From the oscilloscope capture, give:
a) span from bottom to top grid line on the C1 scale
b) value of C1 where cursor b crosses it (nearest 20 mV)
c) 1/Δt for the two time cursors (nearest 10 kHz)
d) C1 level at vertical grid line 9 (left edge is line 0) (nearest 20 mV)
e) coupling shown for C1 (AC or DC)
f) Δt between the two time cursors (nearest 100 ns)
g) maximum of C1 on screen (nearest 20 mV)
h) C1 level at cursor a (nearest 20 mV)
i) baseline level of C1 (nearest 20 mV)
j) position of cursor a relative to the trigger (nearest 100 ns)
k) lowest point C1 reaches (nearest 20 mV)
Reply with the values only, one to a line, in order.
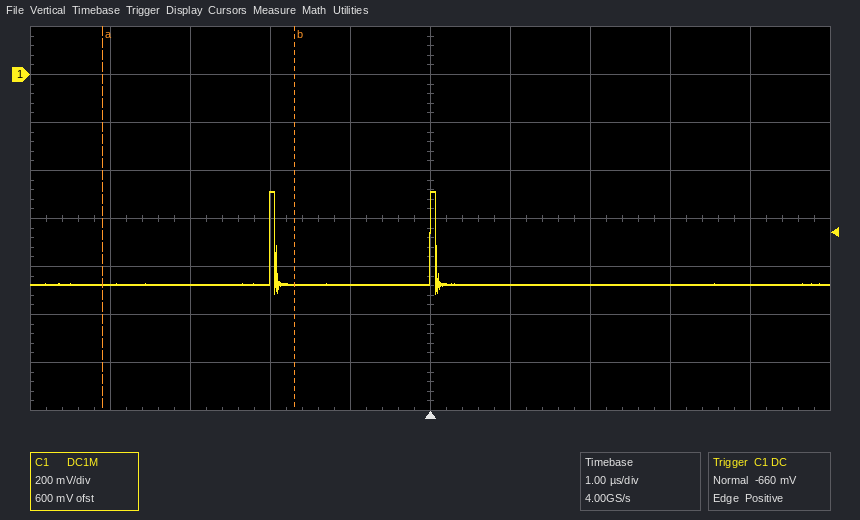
1.6 V
-880 mV
420 kHz
-880 mV
DC
2.4 µs
-480 mV
-880 mV
-880 mV
-4.1 µs
-920 mV
